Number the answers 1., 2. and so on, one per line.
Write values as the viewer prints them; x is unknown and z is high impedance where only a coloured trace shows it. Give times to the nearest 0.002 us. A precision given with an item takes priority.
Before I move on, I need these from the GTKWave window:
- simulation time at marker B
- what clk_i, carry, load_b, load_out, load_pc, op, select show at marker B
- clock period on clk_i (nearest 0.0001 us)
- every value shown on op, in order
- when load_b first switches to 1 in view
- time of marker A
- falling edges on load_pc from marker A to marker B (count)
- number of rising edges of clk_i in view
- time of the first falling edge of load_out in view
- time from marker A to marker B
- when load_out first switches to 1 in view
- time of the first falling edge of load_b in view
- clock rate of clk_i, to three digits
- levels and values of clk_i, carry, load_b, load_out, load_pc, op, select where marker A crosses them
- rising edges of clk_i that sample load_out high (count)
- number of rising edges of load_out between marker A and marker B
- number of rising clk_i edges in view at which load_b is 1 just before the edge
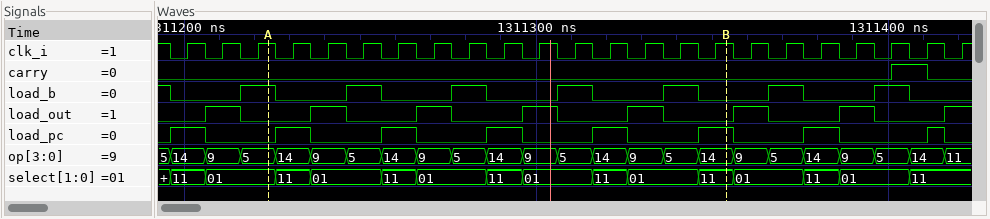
1. 1311.354 us
2. clk_i=1, carry=0, load_b=0, load_out=0, load_pc=1, op=14, select=11
3. 0.01 us
4. 5, 14, 9, 5, 14, 9, 5, 14, 9, 5, 14, 9, 5, 14, 9, 5, 14, 9, 5, 14, 9, 5, 14, 11
5. 1311.216 us
6. 1311.224 us
7. 4
8. 23
9. 1311.216 us
10. 0.13 us
11. 1311.206 us
12. 1311.196 us
13. 100 MHz
14. clk_i=1, carry=0, load_b=1, load_out=0, load_pc=0, op=5, select=01
15. 8
16. 4
17. 7
